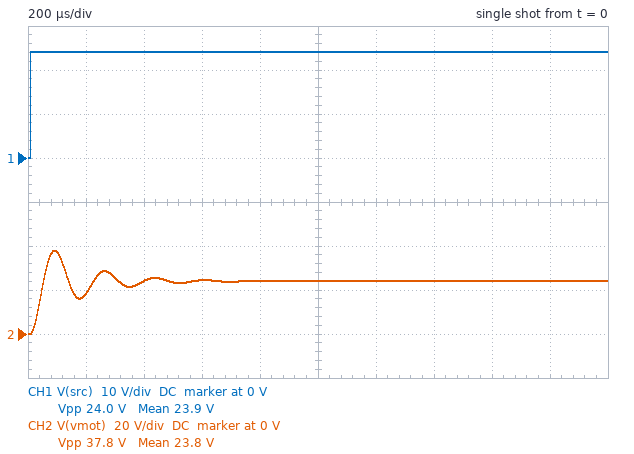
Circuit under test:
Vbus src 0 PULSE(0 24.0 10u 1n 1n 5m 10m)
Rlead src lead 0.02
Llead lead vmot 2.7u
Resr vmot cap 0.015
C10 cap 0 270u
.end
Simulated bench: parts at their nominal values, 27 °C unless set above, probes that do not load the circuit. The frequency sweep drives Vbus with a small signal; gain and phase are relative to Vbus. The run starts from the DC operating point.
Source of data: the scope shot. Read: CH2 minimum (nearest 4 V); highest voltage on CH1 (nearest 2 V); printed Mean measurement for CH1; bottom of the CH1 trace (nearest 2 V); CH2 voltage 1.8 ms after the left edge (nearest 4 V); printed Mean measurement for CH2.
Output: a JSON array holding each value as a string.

["0 V", "24 V", "23.9 V", "0 V", "24 V", "23.8 V"]
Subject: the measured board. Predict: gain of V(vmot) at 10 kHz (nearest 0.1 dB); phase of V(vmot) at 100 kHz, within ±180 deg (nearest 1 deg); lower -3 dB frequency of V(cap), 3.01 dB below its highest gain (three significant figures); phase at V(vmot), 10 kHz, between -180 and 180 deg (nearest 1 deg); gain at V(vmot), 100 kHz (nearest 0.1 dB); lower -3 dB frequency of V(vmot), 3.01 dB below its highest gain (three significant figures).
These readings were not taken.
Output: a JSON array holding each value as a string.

["-5.6 dB", "-110 deg", "4.54 kHz", "-148 deg", "-40.4 dB", "4.55 kHz"]
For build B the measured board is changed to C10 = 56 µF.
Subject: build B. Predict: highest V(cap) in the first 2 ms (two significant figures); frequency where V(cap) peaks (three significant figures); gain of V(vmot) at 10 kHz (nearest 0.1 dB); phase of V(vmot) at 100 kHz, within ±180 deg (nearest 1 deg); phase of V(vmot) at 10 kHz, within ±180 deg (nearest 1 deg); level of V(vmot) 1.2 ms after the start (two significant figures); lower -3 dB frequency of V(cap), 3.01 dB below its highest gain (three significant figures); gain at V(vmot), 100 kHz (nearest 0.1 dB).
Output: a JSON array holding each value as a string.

["43 V", "12.9 kHz", "7.5 dB", "-151 deg", "-14 deg", "24 V", "11.8 kHz", "-34.3 dB"]
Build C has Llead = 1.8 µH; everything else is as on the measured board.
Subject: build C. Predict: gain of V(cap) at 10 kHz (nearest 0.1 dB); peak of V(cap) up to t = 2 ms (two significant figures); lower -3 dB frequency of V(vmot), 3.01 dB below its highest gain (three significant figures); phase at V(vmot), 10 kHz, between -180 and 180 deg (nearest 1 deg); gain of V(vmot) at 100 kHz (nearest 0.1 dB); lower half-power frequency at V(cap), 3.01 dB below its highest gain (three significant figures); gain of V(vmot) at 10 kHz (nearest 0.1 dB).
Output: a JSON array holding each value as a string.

["-0.8 dB", "36 V", "5.08 kHz", "-133 deg", "-36.9 dB", "5.05 kHz", "-0.5 dB"]
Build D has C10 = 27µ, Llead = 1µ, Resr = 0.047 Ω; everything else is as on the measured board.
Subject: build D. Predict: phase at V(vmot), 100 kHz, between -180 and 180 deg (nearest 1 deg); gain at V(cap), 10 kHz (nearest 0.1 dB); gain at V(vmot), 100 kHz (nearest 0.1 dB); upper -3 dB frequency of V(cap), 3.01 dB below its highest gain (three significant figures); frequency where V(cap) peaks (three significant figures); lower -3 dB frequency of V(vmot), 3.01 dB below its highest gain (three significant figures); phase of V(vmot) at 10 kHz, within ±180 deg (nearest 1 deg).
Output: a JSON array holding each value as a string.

["-135 deg", "0.9 dB", "-17.6 dB", "34.7 kHz", "29.7 kHz", "23.8 kHz", "-3 deg"]
